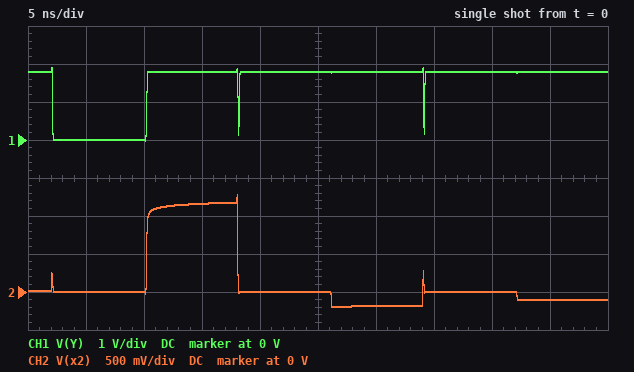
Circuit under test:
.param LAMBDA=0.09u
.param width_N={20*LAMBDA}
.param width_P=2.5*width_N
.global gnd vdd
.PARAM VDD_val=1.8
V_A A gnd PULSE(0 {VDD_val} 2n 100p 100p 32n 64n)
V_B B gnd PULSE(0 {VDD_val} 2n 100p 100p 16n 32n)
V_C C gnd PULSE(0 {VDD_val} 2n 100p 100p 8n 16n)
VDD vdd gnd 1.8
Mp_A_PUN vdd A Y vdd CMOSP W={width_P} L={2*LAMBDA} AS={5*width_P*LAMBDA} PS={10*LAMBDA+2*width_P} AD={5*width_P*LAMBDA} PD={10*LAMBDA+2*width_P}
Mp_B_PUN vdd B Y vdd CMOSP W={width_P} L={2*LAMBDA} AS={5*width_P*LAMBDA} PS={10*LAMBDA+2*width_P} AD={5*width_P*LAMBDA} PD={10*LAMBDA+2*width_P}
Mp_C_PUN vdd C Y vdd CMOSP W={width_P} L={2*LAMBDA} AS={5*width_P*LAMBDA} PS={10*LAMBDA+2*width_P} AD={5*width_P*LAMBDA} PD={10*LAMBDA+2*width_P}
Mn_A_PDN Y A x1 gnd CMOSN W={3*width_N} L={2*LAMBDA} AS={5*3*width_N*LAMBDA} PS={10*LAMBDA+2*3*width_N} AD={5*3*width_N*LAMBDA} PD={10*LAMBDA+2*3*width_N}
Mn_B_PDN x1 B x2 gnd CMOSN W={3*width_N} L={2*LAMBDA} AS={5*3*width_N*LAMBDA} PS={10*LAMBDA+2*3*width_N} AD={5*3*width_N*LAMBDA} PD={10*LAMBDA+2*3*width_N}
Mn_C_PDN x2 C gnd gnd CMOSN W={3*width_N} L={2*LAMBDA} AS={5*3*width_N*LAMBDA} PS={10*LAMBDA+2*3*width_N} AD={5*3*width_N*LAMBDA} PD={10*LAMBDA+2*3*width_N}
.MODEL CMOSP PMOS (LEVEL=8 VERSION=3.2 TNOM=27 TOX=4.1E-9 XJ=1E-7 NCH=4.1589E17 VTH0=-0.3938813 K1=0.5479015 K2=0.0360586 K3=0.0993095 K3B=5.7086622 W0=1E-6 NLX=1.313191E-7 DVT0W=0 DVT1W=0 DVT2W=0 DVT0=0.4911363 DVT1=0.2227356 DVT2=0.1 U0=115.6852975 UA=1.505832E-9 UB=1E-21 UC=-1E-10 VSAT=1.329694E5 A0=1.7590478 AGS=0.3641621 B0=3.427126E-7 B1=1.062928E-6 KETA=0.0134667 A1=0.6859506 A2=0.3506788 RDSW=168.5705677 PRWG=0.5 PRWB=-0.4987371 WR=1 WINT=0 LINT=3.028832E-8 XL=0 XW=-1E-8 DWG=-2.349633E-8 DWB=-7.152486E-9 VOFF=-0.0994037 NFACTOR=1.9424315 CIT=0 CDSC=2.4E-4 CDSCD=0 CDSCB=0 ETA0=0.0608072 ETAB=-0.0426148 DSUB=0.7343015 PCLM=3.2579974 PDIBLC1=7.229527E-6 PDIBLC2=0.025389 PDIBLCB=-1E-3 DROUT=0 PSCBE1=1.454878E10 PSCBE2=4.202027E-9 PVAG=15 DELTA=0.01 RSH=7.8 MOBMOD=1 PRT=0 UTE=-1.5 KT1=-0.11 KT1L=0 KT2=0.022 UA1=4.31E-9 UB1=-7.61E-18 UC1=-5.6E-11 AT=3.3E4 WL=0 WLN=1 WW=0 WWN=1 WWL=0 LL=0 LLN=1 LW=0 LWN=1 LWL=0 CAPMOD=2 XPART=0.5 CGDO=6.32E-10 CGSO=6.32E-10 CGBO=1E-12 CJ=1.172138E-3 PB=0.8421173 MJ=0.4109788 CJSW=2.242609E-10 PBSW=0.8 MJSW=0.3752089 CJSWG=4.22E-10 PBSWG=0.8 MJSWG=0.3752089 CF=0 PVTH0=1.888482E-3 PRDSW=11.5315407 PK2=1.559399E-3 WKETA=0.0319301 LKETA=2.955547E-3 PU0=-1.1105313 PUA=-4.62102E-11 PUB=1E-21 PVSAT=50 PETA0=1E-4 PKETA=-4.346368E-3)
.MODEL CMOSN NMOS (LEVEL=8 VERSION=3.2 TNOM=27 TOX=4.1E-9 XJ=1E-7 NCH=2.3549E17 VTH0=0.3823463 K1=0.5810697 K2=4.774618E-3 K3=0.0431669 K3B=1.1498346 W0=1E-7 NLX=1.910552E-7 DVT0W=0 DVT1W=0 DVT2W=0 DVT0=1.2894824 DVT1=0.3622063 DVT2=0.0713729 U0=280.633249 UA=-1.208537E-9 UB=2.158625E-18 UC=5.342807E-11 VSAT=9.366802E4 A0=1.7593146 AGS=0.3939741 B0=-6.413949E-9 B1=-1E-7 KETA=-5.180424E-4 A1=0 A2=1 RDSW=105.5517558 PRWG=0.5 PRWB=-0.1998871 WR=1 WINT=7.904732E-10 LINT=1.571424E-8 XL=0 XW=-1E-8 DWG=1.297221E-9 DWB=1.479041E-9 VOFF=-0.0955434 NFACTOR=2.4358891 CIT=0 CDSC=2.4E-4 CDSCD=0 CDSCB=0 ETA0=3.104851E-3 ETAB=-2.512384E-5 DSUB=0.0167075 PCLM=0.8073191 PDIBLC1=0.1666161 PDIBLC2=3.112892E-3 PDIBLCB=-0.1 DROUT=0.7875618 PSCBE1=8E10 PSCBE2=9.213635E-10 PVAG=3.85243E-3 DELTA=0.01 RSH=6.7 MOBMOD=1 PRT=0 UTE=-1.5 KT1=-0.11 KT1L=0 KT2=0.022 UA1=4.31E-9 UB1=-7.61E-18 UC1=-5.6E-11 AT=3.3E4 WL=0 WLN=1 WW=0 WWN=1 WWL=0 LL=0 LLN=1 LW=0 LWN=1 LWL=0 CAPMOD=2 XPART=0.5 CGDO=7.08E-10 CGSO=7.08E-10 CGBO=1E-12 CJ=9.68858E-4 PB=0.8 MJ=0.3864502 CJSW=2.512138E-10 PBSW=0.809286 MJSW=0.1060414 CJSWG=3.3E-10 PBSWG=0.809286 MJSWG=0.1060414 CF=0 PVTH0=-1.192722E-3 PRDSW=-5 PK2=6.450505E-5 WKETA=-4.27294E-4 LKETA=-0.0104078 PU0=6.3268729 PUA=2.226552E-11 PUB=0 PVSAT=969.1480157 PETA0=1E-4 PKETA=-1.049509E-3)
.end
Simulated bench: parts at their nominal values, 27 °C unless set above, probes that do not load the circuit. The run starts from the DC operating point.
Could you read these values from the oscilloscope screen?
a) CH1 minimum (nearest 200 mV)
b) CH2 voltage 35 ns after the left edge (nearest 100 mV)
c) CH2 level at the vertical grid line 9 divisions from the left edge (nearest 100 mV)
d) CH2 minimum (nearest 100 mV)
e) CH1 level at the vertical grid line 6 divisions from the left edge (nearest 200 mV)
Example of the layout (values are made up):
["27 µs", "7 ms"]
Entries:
["0 V", "0 V", "-100 mV", "-200 mV", "1.8 V"]
